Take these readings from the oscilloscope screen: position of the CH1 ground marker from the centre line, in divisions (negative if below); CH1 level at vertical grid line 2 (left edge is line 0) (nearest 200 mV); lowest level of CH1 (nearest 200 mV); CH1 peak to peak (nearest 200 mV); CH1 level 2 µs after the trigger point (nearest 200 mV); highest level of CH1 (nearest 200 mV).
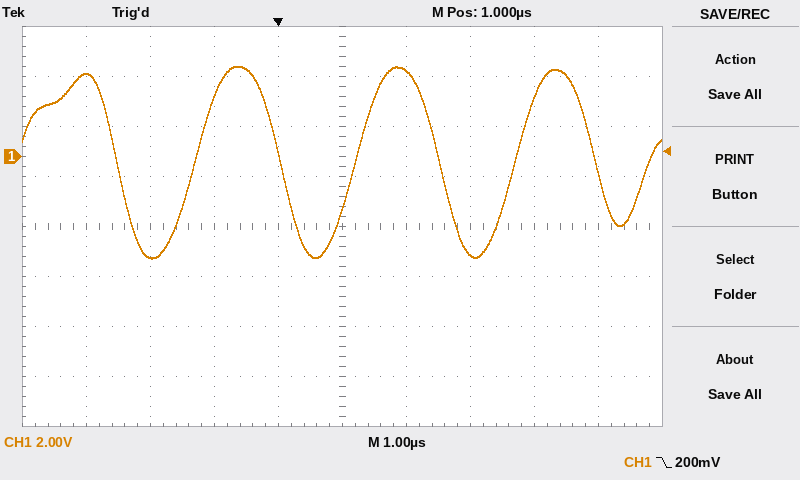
+1.4 div
-4.0 V
-4.0 V
7.6 V
3.4 V
3.6 V
